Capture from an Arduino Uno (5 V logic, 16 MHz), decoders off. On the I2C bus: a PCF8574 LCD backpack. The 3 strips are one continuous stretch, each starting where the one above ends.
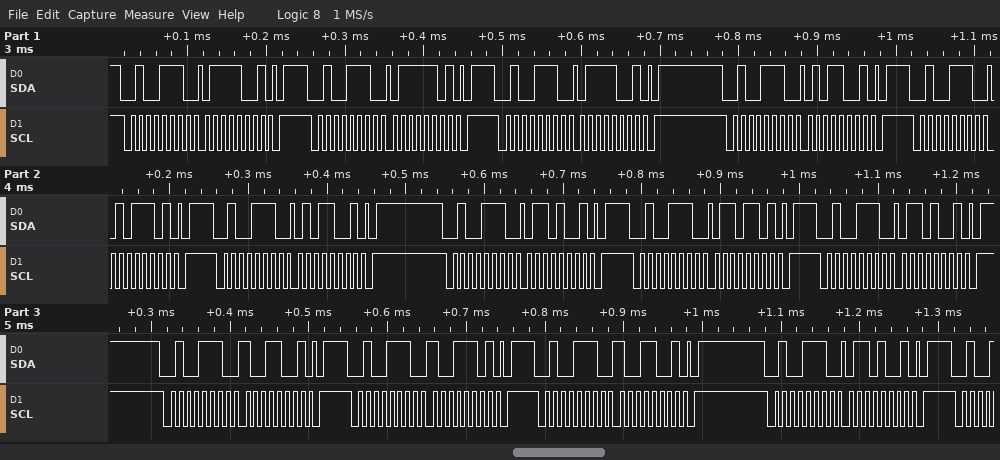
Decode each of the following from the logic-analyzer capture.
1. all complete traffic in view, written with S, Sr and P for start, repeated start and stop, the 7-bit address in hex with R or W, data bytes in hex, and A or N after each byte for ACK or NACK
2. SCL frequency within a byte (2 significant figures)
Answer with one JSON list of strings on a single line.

["S 27W A 79 A P S 27W A 7D A P S 27W A 79 A P S 27W A 59 A P S 27W A 5D A P S 27W A 59 A P S 27W A 69 A P S 27W A 6D A P S 27W A 69 A P S 27W A 99 A P S 27W A 9D A P S 27W A 99 A P S 27W A 69 A P", "100 kHz"]
